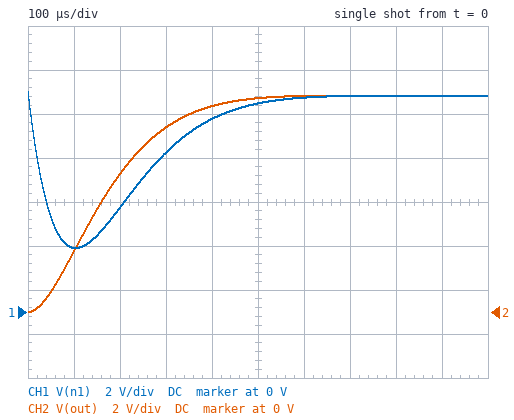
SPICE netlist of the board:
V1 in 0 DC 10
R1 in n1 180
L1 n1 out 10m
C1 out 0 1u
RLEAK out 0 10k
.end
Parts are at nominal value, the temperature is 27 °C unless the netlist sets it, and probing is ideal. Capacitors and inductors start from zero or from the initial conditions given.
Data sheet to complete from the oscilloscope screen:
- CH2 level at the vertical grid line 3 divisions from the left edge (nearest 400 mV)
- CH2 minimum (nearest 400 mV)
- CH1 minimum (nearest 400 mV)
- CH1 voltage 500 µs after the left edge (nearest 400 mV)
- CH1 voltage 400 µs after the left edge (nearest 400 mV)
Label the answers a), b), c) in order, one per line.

a) 8.4 V
b) 0 V
c) 2.8 V
d) 9.6 V
e) 8.8 V
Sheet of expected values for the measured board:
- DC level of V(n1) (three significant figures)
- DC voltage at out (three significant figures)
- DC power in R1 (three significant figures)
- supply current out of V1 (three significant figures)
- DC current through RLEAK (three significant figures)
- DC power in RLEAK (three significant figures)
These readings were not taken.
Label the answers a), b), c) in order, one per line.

a) 9.82 V
b) 9.82 V
c) 174 µW
d) 982 µA
e) 982 µA
f) 9.65 mW
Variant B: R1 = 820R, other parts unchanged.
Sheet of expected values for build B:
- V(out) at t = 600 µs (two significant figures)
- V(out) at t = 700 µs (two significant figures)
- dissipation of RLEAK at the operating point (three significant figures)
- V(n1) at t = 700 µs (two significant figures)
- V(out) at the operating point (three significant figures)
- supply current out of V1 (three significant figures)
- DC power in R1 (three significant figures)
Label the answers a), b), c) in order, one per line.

a) 5.0 V
b) 5.6 V
c) 8.54 mW
d) 5.5 V
e) 9.24 V
f) 924 µA
g) 700 µW
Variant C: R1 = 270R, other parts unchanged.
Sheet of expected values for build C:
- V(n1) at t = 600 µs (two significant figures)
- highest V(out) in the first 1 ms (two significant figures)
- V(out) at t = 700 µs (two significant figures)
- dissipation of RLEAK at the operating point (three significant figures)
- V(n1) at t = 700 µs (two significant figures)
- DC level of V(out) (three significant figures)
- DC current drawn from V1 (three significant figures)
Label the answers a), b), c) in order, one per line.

a) 8.8 V
b) 9.6 V
c) 9.2 V
d) 9.48 mW
e) 9.1 V
f) 9.74 V
g) 974 µA
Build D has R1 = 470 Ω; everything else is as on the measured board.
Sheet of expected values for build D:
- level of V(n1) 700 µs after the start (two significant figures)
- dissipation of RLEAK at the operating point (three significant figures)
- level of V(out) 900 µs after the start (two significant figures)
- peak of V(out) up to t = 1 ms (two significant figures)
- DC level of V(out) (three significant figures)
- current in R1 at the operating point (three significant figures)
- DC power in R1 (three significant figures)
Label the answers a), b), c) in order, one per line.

a) 7.5 V
b) 9.12 mW
c) 8.3 V
d) 8.6 V
e) 9.55 V
f) 955 µA
g) 429 µW
